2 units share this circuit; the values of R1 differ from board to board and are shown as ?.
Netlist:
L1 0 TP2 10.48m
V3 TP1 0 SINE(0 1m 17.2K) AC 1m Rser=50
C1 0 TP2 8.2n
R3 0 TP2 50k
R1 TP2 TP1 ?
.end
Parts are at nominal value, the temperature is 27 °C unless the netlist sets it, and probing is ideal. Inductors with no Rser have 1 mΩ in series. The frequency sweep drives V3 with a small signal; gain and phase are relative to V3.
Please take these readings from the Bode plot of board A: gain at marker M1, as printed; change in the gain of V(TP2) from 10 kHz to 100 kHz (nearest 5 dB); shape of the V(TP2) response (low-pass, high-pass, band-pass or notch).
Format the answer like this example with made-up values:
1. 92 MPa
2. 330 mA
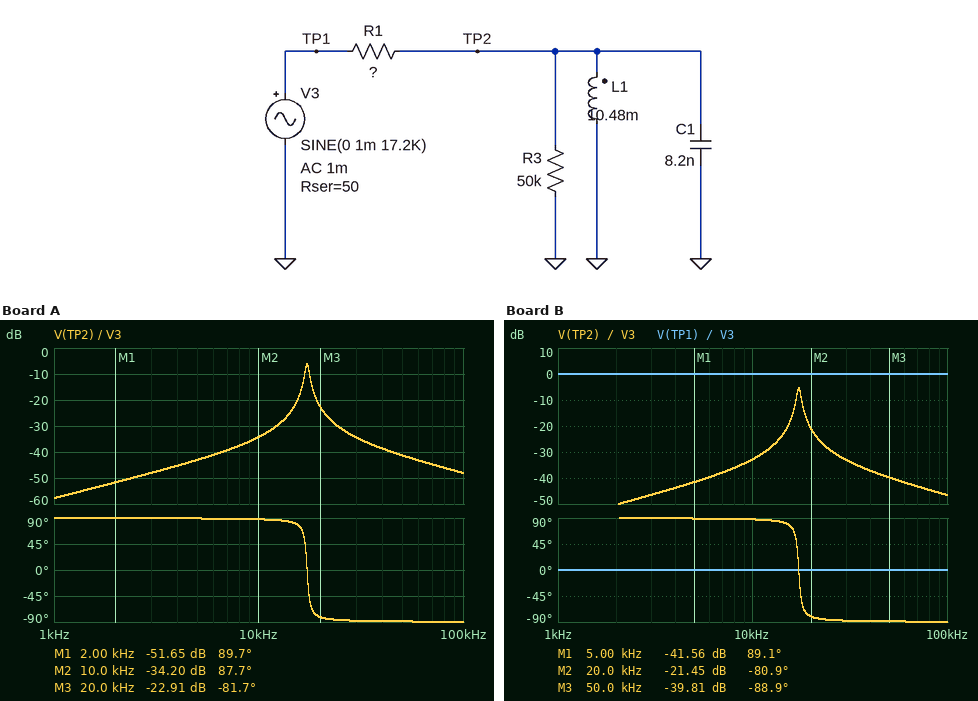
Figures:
1. -51.65 dB
2. -15 dB
3. band-pass
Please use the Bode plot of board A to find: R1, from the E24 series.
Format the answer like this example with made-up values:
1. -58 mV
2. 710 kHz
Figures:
1. 51 kΩ
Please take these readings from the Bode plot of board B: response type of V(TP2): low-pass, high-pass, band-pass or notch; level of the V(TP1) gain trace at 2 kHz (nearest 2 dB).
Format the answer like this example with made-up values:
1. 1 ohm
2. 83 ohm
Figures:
1. band-pass
2. 0 dB
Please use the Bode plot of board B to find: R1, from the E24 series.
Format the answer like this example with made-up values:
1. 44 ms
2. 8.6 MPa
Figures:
1. 43 kΩ
